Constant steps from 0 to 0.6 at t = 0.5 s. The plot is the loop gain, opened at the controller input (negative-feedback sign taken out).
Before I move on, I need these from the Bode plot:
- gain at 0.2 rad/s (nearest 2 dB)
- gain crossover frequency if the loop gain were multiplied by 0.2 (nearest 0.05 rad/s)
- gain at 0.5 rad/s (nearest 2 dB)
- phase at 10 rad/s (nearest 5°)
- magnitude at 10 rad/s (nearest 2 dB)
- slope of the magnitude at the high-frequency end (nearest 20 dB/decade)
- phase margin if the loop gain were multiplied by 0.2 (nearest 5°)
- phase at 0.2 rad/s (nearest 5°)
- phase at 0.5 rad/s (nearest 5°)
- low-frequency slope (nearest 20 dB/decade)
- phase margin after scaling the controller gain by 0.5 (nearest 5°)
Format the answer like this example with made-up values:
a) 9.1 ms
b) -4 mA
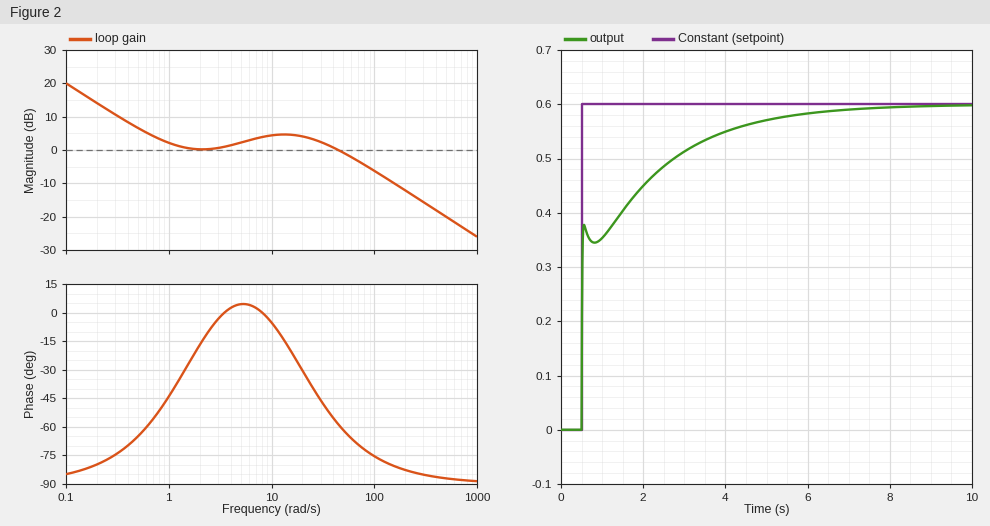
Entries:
a) 14 dB
b) 0.20 rad/s
c) 6 dB
d) -5°
e) 4 dB
f) -20 dB/decade
g) 100°
h) -80°
i) -65°
j) -20 dB/decade
k) 115°
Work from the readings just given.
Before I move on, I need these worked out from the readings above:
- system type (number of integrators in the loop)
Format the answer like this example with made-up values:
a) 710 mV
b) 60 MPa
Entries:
a) 1
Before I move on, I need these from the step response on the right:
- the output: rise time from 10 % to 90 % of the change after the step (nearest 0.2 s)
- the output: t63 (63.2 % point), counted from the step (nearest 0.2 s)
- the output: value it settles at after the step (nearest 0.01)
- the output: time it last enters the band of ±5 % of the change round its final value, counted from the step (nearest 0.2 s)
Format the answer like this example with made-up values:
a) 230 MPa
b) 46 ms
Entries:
a) 3.2 s
b) 0.8 s
c) 0.60
d) 4.4 s
